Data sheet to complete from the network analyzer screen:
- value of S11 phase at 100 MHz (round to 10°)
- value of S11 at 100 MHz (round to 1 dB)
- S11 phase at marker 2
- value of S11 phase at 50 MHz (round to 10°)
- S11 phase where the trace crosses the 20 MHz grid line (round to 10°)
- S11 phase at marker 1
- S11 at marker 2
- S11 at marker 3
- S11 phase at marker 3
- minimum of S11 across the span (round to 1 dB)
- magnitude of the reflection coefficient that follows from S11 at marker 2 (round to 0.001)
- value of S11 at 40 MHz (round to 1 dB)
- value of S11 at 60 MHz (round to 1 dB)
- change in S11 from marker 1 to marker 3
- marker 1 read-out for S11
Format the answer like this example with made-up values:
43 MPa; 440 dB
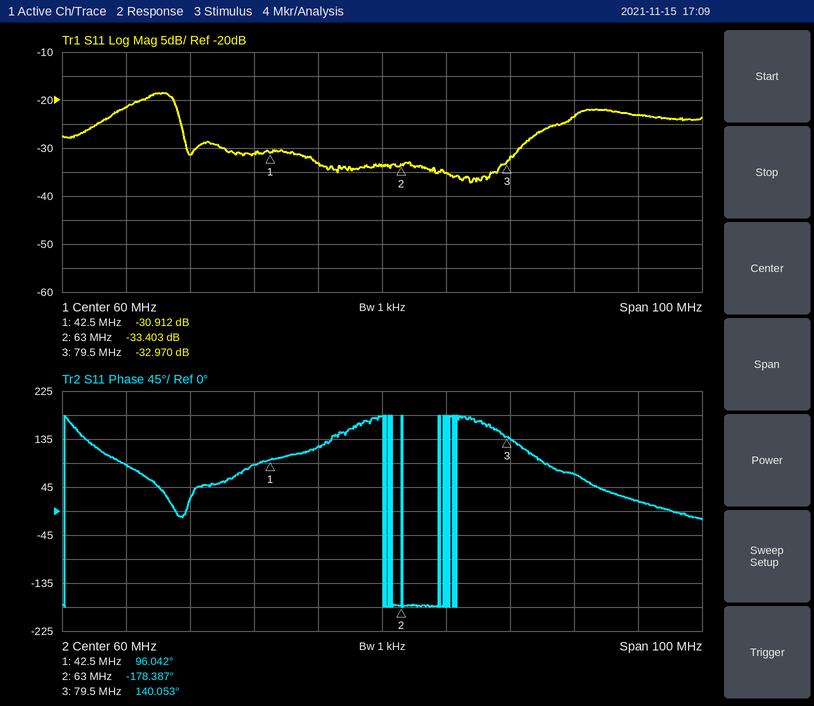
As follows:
20°; -23 dB; -178.387°; 120°; 90°; 96.042°; -33.403 dB; -32.970 dB; 140.053°; -37 dB; 0.021; -31 dB; -34 dB; -2.058 dB; -30.912 dB
